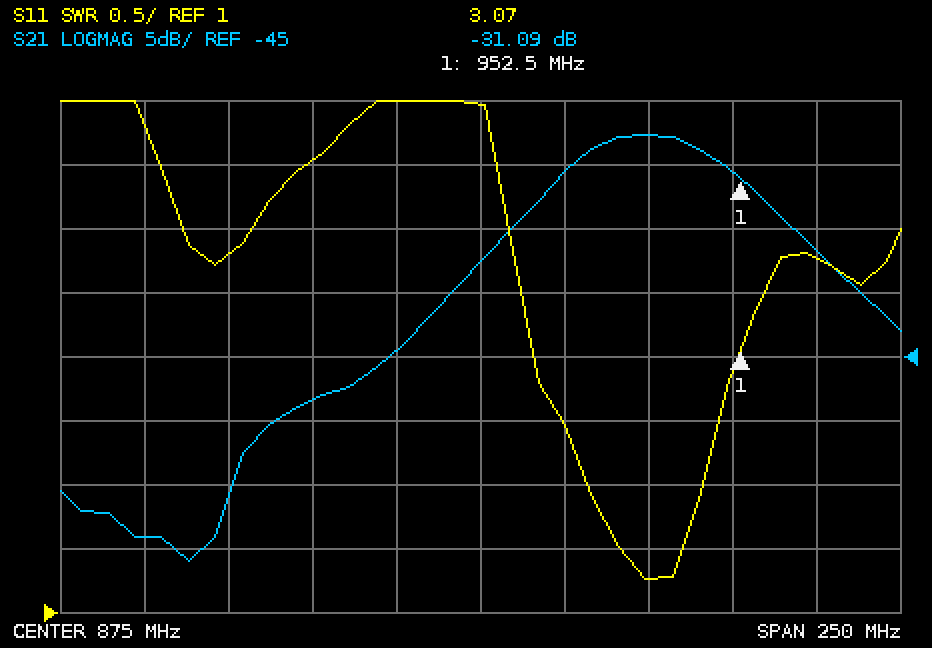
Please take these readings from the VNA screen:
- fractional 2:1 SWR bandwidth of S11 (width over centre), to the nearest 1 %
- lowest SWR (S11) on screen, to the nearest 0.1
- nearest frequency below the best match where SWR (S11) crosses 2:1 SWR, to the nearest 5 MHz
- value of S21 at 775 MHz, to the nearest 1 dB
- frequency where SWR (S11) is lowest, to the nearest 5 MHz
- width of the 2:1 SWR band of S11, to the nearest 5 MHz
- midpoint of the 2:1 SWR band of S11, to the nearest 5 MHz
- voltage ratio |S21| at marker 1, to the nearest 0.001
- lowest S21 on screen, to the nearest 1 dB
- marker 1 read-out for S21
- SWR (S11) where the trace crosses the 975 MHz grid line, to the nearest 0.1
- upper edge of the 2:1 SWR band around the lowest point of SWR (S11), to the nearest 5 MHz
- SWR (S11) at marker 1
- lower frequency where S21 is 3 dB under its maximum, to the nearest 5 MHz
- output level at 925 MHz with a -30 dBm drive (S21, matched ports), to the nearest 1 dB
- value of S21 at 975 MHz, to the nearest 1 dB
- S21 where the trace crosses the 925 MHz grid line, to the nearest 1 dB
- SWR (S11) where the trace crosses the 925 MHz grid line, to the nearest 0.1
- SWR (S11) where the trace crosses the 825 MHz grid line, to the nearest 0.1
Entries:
4 %
1.3
905 MHz
-59 dB
925 MHz
35 MHz
925 MHz
0.028
-61 dB
-31.09 dB
3.8
940 MHz
3.07
900 MHz
-58 dBm
-37 dB
-28 dB
1.3
4.5
